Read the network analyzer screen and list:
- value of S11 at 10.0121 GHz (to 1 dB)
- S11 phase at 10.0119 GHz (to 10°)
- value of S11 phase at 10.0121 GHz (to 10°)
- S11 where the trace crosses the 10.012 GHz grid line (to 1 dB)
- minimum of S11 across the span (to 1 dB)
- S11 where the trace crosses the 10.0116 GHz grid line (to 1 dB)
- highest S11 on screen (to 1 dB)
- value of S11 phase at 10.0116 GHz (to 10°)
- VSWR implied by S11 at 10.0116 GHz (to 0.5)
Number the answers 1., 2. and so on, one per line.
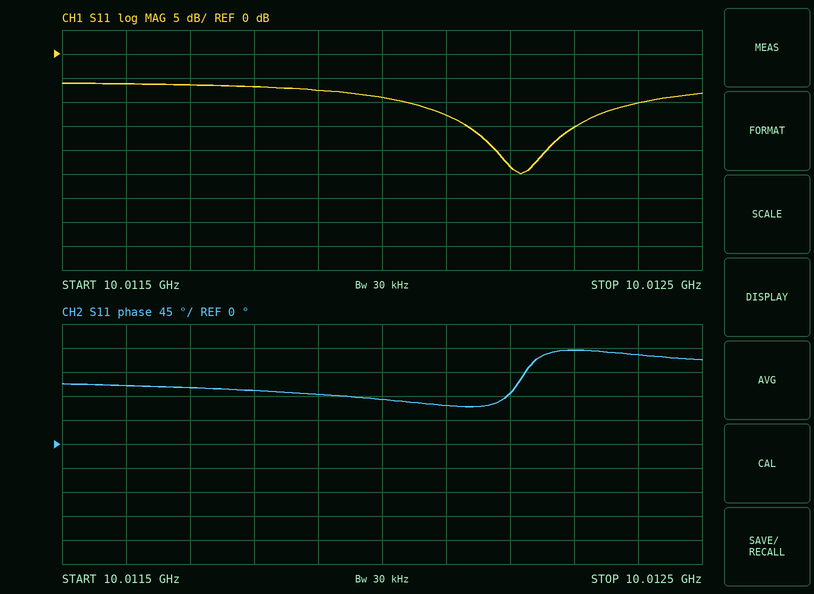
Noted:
1. -13 dB
2. 90°
3. 70°
4. -9 dB
5. -25 dB
6. -6 dB
7. -6 dB
8. 110°
9. 3.0
